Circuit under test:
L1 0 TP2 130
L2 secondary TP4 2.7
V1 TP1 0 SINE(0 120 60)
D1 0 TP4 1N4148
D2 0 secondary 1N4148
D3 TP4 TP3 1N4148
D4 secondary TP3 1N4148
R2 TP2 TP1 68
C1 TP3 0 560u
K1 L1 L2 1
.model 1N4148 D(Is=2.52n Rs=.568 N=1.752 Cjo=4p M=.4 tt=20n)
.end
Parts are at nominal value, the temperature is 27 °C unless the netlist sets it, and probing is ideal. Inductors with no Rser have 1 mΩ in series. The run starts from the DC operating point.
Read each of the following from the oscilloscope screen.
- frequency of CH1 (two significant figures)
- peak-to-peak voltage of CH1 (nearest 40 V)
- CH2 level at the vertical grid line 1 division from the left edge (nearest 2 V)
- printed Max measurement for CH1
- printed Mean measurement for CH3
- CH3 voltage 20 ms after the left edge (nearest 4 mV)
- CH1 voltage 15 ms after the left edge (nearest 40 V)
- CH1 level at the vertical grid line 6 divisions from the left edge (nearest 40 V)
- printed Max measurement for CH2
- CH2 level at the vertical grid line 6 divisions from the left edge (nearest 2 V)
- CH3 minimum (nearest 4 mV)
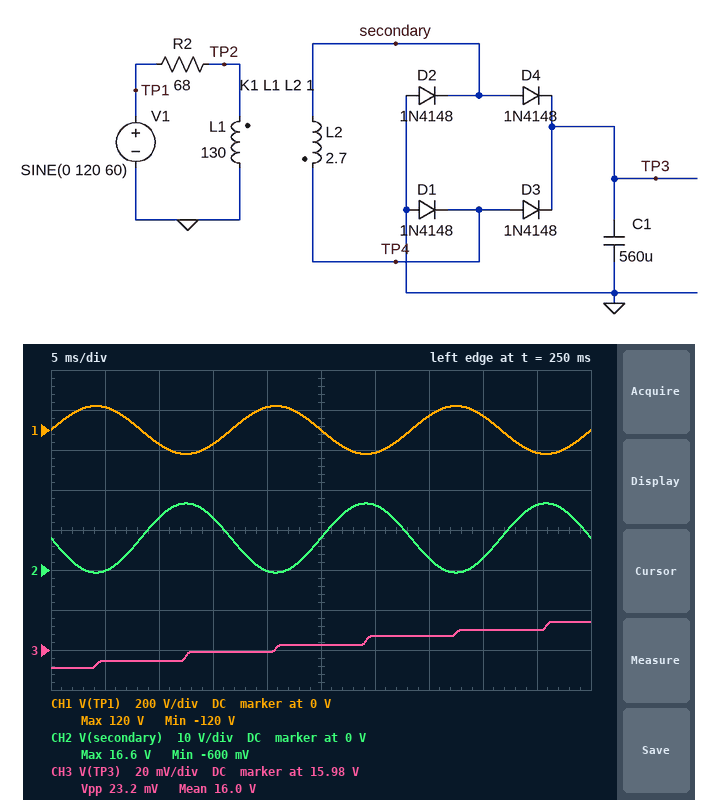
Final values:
60 Hz
240 V
0 V
120 V
16.0 V
15.980 V
-80 V
-120 V
16.6 V
16 V
15.972 V
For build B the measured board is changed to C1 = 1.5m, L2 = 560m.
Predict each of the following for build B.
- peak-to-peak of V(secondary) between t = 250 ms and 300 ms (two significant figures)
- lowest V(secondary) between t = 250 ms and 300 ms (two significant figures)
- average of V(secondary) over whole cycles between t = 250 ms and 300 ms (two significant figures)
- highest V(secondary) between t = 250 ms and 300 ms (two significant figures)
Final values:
7.9 V
-680 mV
3.3 V
7.2 V
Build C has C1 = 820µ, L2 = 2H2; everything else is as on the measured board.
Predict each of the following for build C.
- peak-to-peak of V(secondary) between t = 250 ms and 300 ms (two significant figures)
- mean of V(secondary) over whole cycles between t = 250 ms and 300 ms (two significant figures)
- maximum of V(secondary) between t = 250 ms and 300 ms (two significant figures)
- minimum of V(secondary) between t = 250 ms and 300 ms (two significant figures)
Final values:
16 V
7.1 V
15 V
-670 mV
